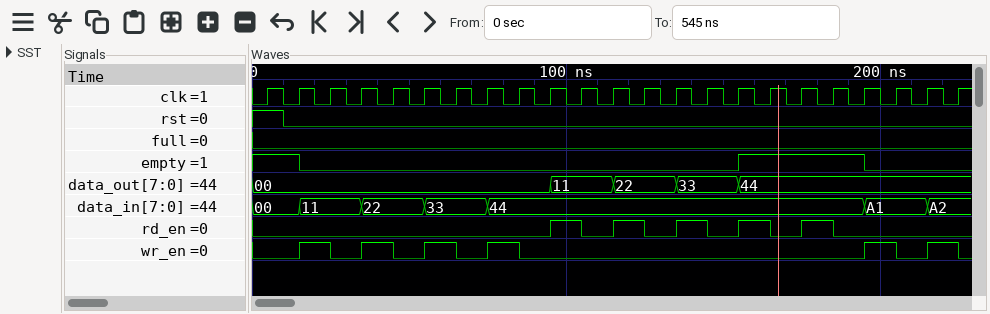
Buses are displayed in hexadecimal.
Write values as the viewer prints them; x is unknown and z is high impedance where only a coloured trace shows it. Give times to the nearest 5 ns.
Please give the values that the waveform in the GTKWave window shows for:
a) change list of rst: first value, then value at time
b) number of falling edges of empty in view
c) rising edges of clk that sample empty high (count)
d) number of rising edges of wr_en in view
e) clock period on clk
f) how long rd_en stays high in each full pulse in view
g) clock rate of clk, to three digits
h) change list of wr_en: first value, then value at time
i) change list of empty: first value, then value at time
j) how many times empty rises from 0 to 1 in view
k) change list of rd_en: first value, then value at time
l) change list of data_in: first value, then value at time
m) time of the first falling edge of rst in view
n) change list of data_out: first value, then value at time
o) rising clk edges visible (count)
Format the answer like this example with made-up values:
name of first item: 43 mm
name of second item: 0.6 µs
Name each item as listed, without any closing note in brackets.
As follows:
change list of rst: first value, then value at time: 1, 0 at 10 ns
number of falling edges of empty in view: 2
rising edges of clk that sample empty high: 6
number of rising edges of wr_en in view: 6
clock period on clk: 10 ns
how long rd_en stays high in each full pulse in view: 10 ns, 10 ns, 10 ns, 10 ns, 10 ns
clock rate of clk, to three digits: 100 MHz
change list of wr_en: first value, then value at time: 0, 1 at 15 ns, 0 at 25 ns, 1 at 35 ns, 0 at 45 ns, 1 at 55 ns, 0 at 65 ns, 1 at 75 ns, 0 at 85 ns, 1 at 195 ns, 0 at 205 ns, 1 at 215 ns, 0 at 225 ns
change list of empty: first value, then value at time: 1, 0 at 15 ns, 1 at 155 ns, 0 at 195 ns
how many times empty rises from 0 to 1 in view: 1
change list of rd_en: first value, then value at time: 0, 1 at 95 ns, 0 at 105 ns, 1 at 115 ns, 0 at 125 ns, 1 at 135 ns, 0 at 145 ns, 1 at 155 ns, 0 at 165 ns, 1 at 175 ns, 0 at 185 ns
change list of data_in: first value, then value at time: 00, 11 at 15 ns, 22 at 35 ns, 33 at 55 ns, 44 at 75 ns, A1 at 195 ns, A2 at 215 ns
time of the first falling edge of rst in view: 10 ns
change list of data_out: first value, then value at time: 00, 11 at 95 ns, 22 at 115 ns, 33 at 135 ns, 44 at 155 ns
rising clk edges visible: 23
